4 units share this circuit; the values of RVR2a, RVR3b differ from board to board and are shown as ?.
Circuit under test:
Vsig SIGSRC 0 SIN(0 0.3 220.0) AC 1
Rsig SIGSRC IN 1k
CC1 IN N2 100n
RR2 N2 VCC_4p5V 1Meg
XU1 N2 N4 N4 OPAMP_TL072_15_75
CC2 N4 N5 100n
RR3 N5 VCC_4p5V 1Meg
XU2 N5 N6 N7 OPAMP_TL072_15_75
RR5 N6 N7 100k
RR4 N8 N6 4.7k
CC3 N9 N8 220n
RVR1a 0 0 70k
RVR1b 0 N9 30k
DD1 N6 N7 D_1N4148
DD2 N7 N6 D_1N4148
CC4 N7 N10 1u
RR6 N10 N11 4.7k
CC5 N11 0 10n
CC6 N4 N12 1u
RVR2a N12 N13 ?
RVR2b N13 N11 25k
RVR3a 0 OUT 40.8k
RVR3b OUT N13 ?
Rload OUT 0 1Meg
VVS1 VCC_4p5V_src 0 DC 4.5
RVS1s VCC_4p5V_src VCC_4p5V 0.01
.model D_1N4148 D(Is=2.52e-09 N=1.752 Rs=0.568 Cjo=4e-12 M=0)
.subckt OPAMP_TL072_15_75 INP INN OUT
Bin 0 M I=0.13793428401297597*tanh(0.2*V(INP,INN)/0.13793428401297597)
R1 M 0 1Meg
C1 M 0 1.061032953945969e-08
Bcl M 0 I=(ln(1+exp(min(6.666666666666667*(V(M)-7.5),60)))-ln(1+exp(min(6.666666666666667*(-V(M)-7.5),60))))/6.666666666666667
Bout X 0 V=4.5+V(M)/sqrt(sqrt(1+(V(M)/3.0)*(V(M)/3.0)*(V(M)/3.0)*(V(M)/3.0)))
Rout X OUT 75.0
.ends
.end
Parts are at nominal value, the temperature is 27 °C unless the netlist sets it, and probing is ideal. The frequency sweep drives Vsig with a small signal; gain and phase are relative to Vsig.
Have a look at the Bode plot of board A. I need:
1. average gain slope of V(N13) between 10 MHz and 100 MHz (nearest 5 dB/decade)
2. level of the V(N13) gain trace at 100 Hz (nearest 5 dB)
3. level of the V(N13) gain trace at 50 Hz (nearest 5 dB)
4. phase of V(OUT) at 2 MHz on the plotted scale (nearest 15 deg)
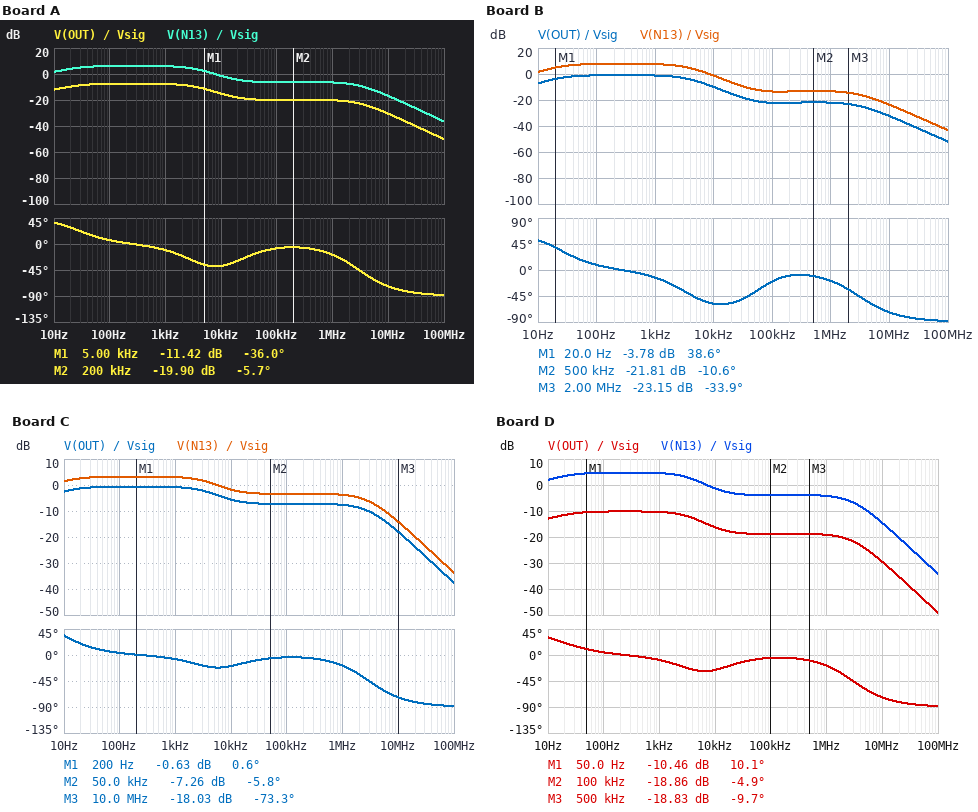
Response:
-20 dB/decade
5 dB
5 dB
-30 deg
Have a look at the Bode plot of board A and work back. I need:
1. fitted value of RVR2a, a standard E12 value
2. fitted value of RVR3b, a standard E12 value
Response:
22 kΩ
150 kΩ
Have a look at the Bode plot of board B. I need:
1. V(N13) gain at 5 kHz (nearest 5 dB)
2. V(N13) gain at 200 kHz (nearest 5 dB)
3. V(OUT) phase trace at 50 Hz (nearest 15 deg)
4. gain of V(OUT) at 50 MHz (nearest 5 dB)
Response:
5 dB
-15 dB
15 deg
-45 dB
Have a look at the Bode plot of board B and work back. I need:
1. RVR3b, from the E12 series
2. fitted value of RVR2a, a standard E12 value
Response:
68 kΩ
68 kΩ
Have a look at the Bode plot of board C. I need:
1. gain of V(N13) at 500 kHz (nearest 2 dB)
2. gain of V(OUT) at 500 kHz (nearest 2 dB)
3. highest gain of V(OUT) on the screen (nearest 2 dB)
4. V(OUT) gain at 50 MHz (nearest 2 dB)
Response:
-4 dB
-8 dB
0 dB
-32 dB
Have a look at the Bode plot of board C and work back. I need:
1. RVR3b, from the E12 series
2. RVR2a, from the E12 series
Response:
22 kΩ
8.2 kΩ
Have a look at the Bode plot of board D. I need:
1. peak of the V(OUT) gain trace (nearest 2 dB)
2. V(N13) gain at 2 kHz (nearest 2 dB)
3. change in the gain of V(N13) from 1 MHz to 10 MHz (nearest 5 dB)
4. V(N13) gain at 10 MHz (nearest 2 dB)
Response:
-10 dB
4 dB
-10 dB
-14 dB
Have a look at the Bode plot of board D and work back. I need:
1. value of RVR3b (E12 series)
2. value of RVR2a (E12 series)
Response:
180 kΩ
12 kΩ
